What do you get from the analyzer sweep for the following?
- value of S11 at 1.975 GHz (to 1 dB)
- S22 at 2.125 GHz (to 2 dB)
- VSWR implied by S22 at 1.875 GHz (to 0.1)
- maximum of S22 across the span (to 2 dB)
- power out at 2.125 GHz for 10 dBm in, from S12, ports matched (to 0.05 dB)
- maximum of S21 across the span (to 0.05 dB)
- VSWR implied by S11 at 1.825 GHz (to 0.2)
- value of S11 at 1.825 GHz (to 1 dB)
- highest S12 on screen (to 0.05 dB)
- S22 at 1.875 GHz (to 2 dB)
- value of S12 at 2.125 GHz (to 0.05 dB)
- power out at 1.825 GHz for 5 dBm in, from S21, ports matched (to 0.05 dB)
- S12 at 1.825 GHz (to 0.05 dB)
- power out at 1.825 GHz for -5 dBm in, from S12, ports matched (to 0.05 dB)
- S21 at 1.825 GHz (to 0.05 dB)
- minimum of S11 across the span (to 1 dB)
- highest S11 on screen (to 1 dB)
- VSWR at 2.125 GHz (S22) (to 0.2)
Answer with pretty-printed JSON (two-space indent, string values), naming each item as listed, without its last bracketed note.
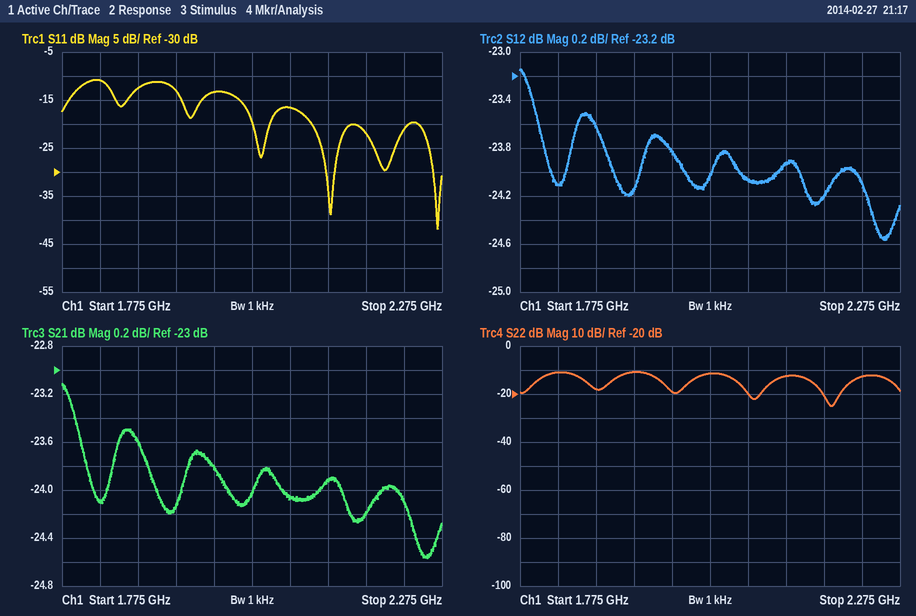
{
  "value of S11 at 1.975 GHz": "-13 dB",
  "S22 at 2.125 GHz": "-12 dB",
  "VSWR implied by S22 at 1.875 GHz": "1.3",
  "maximum of S22 across the span": "-10 dB",
  "power out at 2.125 GHz for 10 dBm in, from S12, ports matched": "-13.95 dBm",
  "maximum of S21 across the span": "-23.10 dB",
  "VSWR implied by S11 at 1.825 GHz": "1.8",
  "value of S11 at 1.825 GHz": "-11 dB",
  "highest S12 on screen": "-23.15 dB",
  "S22 at 1.875 GHz": "-18 dB",
  "value of S12 at 2.125 GHz": "-23.95 dB",
  "power out at 1.825 GHz for 5 dBm in, from S21, ports matched": "-19.10 dBm",
  "S12 at 1.825 GHz": "-24.10 dB",
  "power out at 1.825 GHz for -5 dBm in, from S12, ports matched": "-29.10 dBm",
  "S21 at 1.825 GHz": "-24.10 dB",
  "minimum of S11 across the span": "-42 dB",
  "highest S11 on screen": "-11 dB",
  "VSWR at 2.125 GHz (S22)": "1.6"
}
